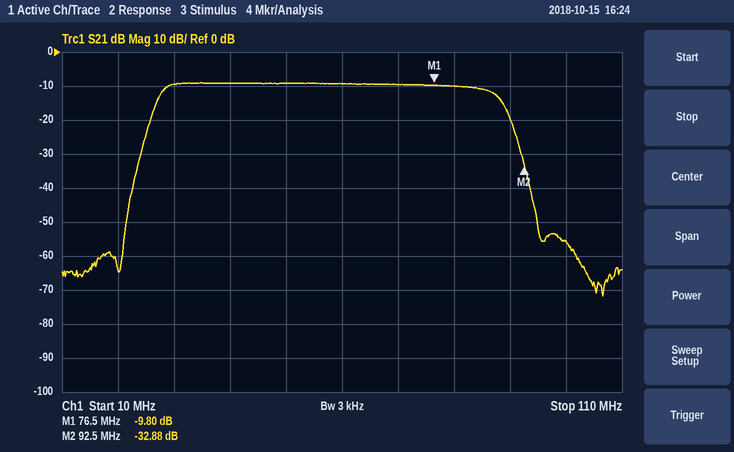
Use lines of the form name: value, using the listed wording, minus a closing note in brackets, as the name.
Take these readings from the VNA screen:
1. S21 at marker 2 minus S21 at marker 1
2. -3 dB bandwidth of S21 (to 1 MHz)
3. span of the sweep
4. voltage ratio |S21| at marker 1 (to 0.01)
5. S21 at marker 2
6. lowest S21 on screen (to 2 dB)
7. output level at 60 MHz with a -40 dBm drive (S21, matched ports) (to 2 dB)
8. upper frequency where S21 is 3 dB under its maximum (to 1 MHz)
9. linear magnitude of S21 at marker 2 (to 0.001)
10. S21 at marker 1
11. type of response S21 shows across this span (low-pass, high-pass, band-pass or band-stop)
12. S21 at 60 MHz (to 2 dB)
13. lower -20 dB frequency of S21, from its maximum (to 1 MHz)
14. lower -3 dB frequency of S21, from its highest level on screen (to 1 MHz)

S21 at marker 2 minus S21 at marker 1: -23.08 dB
-3 dB bandwidth of S21: 59 MHz
span of the sweep: 100 MHz
voltage ratio |S21| at marker 1: 0.32
S21 at marker 2: -32.88 dB
lowest S21 on screen: -72 dB
output level at 60 MHz with a -40 dBm drive (S21, matched ports): -50 dBm
upper frequency where S21 is 3 dB under its maximum: 87 MHz
linear magnitude of S21 at marker 2: 0.023
S21 at marker 1: -9.80 dB
type of response S21 shows across this span: band-pass
S21 at 60 MHz: -10 dB
lower -20 dB frequency of S21, from its maximum: 24 MHz
lower -3 dB frequency of S21, from its highest level on screen: 28 MHz
